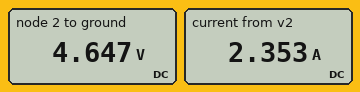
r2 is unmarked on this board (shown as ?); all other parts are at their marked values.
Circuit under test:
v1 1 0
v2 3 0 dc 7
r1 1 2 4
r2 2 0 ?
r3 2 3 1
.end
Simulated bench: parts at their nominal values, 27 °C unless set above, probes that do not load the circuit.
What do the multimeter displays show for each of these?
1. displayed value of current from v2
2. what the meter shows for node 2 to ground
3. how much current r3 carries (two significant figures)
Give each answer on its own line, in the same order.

2.353 A
4.647 V
2.4 A
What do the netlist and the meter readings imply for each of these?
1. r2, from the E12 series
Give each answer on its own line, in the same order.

3.9 Ω
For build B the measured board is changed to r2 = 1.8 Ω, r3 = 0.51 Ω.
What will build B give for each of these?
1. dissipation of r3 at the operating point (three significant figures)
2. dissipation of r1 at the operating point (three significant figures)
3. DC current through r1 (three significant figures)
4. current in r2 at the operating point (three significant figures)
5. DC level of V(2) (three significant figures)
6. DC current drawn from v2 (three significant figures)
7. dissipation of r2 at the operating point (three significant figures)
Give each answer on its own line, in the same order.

8.15 W
6.15 W
1.24 A
2.76 A
4.96 V
4.00 A
13.7 W
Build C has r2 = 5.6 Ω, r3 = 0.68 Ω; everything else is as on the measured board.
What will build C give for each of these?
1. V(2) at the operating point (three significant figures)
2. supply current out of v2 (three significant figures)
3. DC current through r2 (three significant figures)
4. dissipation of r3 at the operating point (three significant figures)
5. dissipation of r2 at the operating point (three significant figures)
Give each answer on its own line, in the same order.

5.42 V
2.32 A
968 mA
3.67 W
5.25 W
